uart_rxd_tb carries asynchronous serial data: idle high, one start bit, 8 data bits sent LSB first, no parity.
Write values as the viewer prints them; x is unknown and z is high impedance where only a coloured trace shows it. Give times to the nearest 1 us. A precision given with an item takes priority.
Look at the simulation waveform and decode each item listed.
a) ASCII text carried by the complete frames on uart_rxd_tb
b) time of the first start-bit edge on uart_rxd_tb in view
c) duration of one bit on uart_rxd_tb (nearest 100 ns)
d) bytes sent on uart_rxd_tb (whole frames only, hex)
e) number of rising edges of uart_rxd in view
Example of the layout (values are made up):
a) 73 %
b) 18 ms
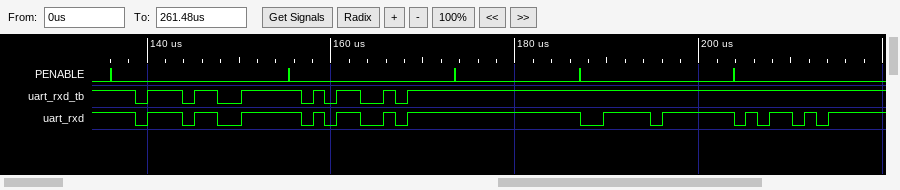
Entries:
a) "7M"
b) 139 us
c) 1300 ns
d) 37, 4D
e) 13
